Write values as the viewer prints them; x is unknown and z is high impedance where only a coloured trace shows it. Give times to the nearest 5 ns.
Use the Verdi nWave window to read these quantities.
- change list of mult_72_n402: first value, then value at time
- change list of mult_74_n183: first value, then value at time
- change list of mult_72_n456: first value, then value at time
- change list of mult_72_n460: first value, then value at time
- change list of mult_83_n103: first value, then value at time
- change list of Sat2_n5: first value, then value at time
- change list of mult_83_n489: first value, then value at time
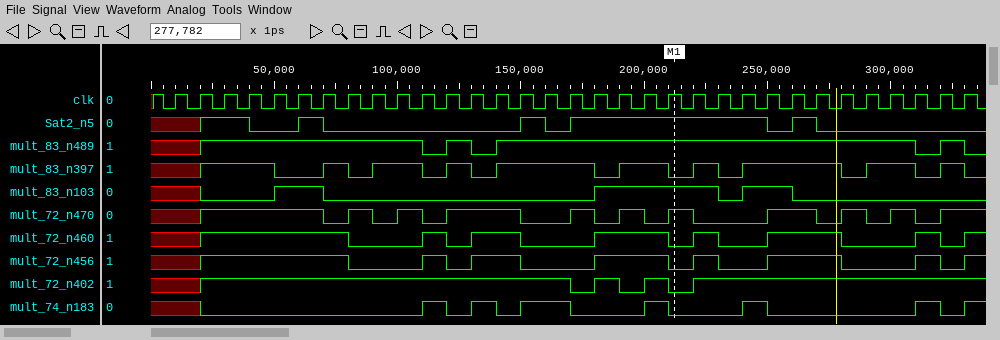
x, 1 at 20 ns, 0 at 170 ns, 1 at 180 ns, 0 at 190 ns, 1 at 200 ns, 0 at 210 ns, 1 at 220 ns
x, 0 at 20 ns, 1 at 110 ns, 0 at 120 ns, 1 at 130 ns, 0 at 140 ns, 1 at 150 ns, 0 at 170 ns, 1 at 200 ns, 0 at 210 ns, 1 at 240 ns, 0 at 250 ns, 1 at 310 ns, 0 at 320 ns, 1 at 330 ns
x, 1 at 20 ns, 0 at 80 ns, 1 at 110 ns, 0 at 120 ns, 1 at 130 ns, 0 at 150 ns, 1 at 180 ns, 0 at 210 ns, 1 at 220 ns, 0 at 230 ns, 1 at 250 ns, 0 at 280 ns, 1 at 310 ns, 0 at 320 ns, 1 at 330 ns
x, 1 at 20 ns, 0 at 80 ns, 1 at 110 ns, 0 at 120 ns, 1 at 130 ns, 0 at 150 ns, 1 at 180 ns, 0 at 210 ns, 1 at 220 ns, 0 at 230 ns, 1 at 250 ns, 0 at 280 ns, 1 at 310 ns, 0 at 320 ns, 1 at 330 ns
x, 0 at 20 ns, 1 at 50 ns, 0 at 70 ns, 1 at 180 ns, 0 at 230 ns, 1 at 240 ns, 0 at 260 ns
x, 1 at 20 ns, 0 at 40 ns, 1 at 60 ns, 0 at 70 ns, 1 at 150 ns, 0 at 160 ns, 1 at 170 ns, 0 at 250 ns, 1 at 260 ns, 0 at 270 ns
x, 1 at 20 ns, 0 at 110 ns, 1 at 120 ns, 0 at 130 ns, 1 at 140 ns, 0 at 310 ns, 1 at 320 ns, 0 at 330 ns
